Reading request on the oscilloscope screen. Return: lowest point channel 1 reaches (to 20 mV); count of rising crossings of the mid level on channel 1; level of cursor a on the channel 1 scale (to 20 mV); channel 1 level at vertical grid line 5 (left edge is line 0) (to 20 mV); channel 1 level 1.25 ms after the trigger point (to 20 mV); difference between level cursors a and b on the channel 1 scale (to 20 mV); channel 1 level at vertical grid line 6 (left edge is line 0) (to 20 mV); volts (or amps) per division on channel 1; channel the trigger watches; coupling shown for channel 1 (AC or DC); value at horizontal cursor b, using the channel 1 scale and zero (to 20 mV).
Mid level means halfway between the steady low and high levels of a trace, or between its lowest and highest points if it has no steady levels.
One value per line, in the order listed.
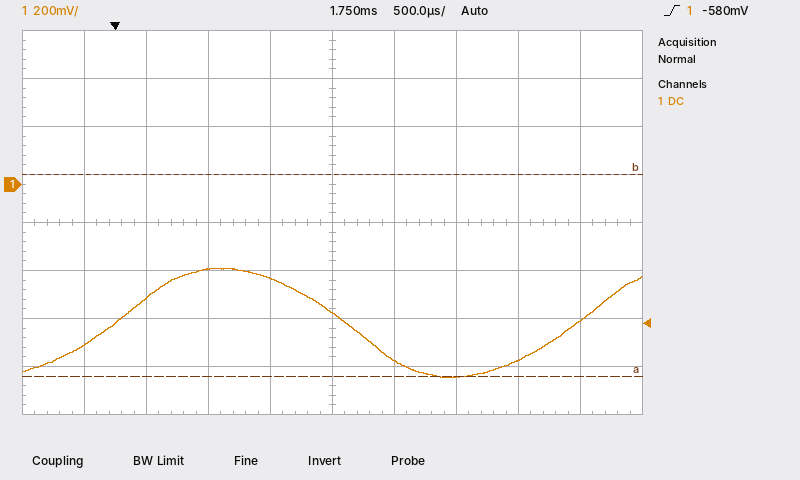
-800 mV
2
-800 mV
-540 mV
-400 mV
840 mV
-740 mV
200 mV
channel 1
DC
40 mV
